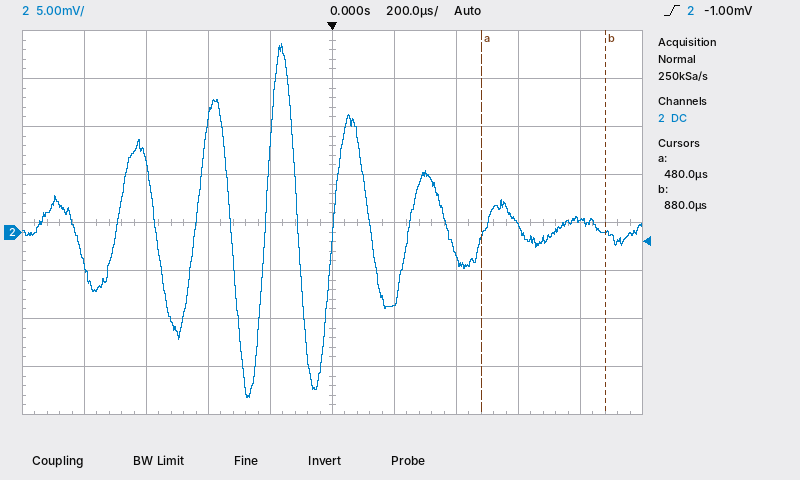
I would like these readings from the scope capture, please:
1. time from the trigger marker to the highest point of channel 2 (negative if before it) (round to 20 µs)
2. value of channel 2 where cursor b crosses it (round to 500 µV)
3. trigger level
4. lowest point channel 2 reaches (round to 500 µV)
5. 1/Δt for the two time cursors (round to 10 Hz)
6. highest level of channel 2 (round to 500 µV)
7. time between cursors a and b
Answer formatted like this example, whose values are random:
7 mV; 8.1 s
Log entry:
-160 µs; 0.0 mV; -1.00 mV; -17.0 mV; 2.50 kHz; 19.5 mV; 400 µs
